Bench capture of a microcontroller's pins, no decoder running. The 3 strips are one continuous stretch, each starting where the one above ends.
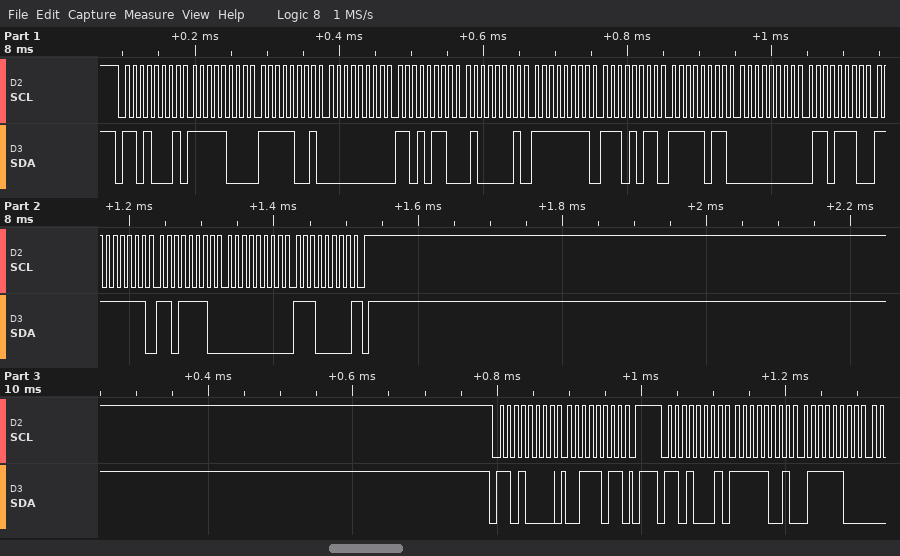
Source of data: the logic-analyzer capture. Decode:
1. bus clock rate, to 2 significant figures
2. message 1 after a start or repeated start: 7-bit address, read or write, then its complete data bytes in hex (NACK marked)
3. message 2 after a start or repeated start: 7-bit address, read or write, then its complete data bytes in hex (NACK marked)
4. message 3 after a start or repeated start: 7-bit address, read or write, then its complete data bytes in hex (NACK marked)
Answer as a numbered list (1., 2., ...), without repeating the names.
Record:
1. 100 kHz
2. 0x68 read: F8 F9 00 D6 41 FF EB FB 00 6E FF DE 00 E0 NACK
3. 0x68 write: 3B
4. 0x68 read: F9 7C
